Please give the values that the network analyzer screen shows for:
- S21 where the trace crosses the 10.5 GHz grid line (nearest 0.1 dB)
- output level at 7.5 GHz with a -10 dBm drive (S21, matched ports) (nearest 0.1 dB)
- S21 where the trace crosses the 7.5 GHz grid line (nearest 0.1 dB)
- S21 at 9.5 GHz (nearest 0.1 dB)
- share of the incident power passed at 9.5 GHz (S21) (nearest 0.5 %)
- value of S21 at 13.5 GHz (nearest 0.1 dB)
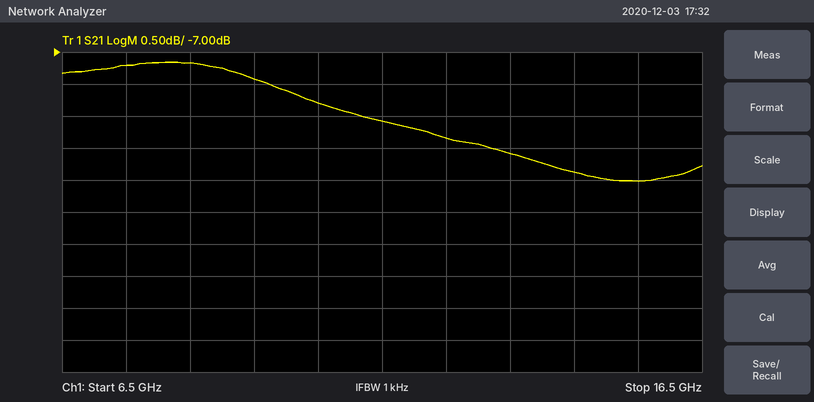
-7.8 dB
-17.2 dBm
-7.2 dB
-7.4 dB
18.0 %
-8.6 dB
